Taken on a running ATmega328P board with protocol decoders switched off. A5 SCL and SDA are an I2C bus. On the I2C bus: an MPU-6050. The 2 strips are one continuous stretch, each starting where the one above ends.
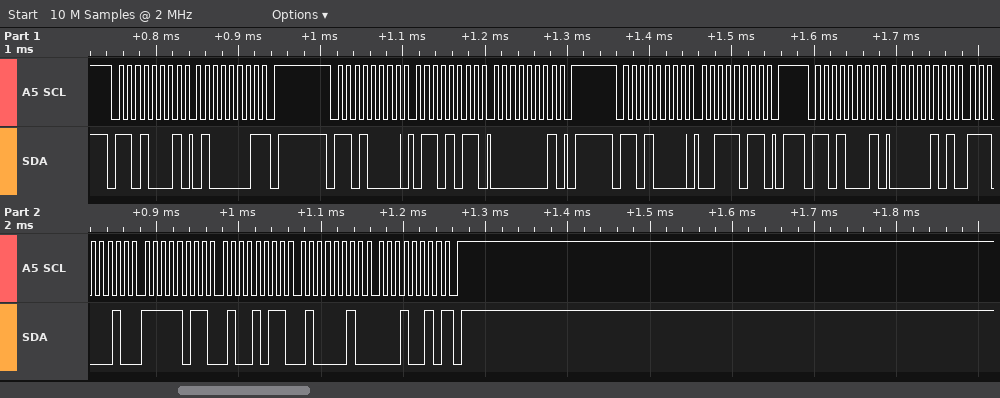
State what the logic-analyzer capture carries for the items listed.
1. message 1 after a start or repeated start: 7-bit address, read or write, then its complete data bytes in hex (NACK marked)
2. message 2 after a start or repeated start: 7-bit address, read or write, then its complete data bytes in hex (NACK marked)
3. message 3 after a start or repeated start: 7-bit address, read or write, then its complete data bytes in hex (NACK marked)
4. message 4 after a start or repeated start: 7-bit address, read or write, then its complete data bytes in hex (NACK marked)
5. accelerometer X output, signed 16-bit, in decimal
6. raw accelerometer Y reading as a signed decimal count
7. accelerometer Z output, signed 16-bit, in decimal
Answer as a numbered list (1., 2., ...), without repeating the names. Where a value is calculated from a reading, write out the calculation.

1. 0x68 read: 41 NACK
2. 0x68 write: 6B 01
3. 0x68 write: 3B
4. 0x68 read: 05 E2 FB 4B 42 12 NACK
5. 0x05E2 = 1506
6. 0xFB4B = -1205
7. 0x4212 = 16914
